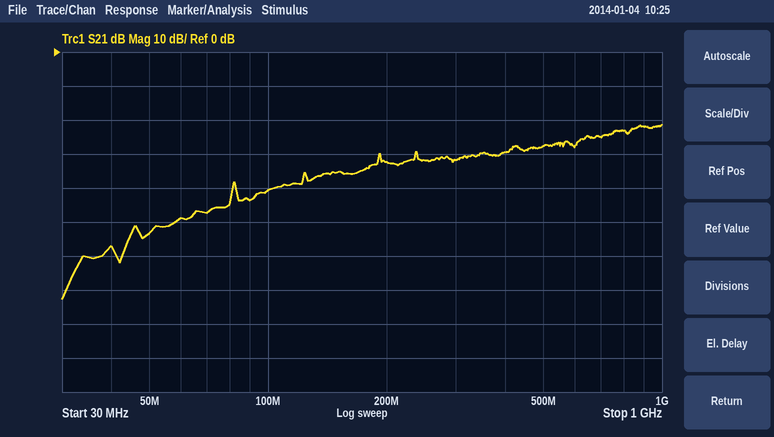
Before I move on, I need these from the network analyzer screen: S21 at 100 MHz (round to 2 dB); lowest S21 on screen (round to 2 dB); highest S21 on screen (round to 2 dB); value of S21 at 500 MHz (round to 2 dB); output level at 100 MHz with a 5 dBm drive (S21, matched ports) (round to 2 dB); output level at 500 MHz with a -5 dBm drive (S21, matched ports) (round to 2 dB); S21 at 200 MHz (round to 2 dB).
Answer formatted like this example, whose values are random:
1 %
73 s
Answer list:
-40 dB
-72 dB
-22 dB
-28 dB
-36 dBm
-32 dBm
-32 dB
